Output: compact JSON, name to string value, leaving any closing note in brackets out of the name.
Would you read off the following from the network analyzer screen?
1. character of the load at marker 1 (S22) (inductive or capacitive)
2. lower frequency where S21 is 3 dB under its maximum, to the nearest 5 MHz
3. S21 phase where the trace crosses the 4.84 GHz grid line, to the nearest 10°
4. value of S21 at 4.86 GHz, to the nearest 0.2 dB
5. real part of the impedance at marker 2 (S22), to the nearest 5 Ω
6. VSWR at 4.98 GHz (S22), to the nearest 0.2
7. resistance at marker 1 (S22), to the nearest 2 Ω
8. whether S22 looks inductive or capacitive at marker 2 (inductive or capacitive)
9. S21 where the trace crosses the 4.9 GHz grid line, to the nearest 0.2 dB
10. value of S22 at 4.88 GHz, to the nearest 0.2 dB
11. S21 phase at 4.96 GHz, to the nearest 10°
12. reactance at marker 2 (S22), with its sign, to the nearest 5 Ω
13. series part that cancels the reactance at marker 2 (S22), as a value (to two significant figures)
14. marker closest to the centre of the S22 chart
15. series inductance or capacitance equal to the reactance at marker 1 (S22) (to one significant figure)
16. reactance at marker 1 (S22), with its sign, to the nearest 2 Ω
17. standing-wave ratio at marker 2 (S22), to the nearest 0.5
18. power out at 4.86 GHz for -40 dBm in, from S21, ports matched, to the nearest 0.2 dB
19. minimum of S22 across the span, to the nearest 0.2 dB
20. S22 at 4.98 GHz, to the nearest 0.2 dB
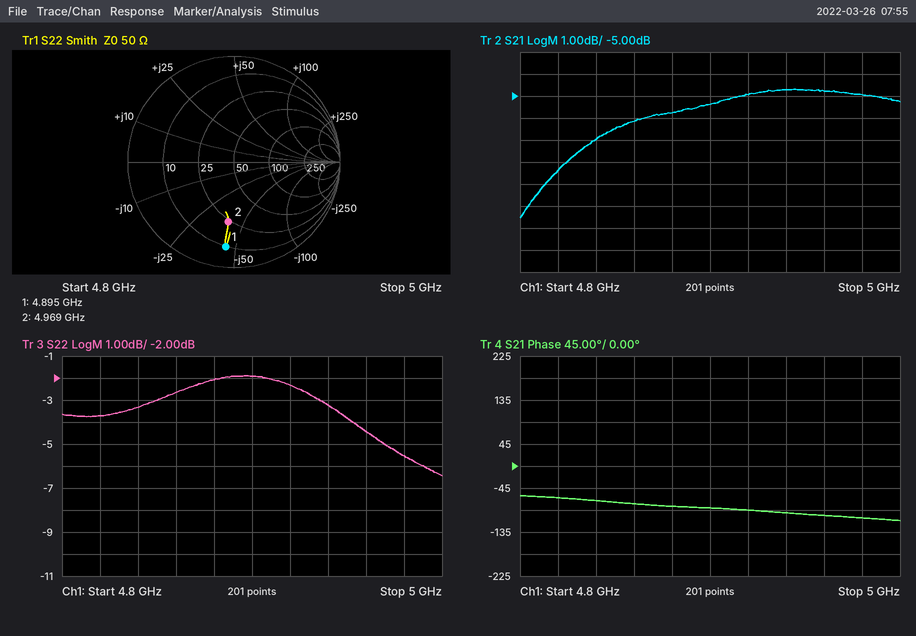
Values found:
{"character of the load at marker 1 (S22)": "capacitive", "lower frequency where S21 is 3 dB under its maximum, to the nearest 5 MHz": "4.830 GHz", "S21 phase where the trace crosses the 4.84 GHz grid line, to the nearest 10°": "-70°", "value of S21 at 4.86 GHz, to the nearest 0.2 dB": "-6.2 dB", "real part of the impedance at marker 2 (S22), to the nearest 5 Ω": "25 Ω", "VSWR at 4.98 GHz (S22), to the nearest 0.2": "3.2", "resistance at marker 1 (S22), to the nearest 2 Ω": "10 Ω", "whether S22 looks inductive or capacitive at marker 2": "capacitive", "S21 where the trace crosses the 4.9 GHz grid line, to the nearest 0.2 dB": "-5.4 dB", "value of S22 at 4.88 GHz, to the nearest 0.2 dB": "-2.0 dB", "S21 phase at 4.96 GHz, to the nearest 10°": "-100°", "reactance at marker 2 (S22), with its sign, to the nearest 5 Ω": "-40 Ω", "series part that cancels the reactance at marker 2 (S22), as a value": "1.3 nH", "marker closest to the centre of the S22 chart": "marker 2", "series inductance or capacitance equal to the reactance at marker 1 (S22)": "700 fF", "reactance at marker 1 (S22), with its sign, to the nearest 2 Ω": "-44 Ω", "standing-wave ratio at marker 2 (S22), to the nearest 0.5": "3.5", "power out at 4.86 GHz for -40 dBm in, from S21, ports matched, to the nearest 0.2 dB": "-46.2 dBm", "minimum of S22 across the span, to the nearest 0.2 dB": "-6.4 dB", "S22 at 4.98 GHz, to the nearest 0.2 dB": "-5.6 dB"}
